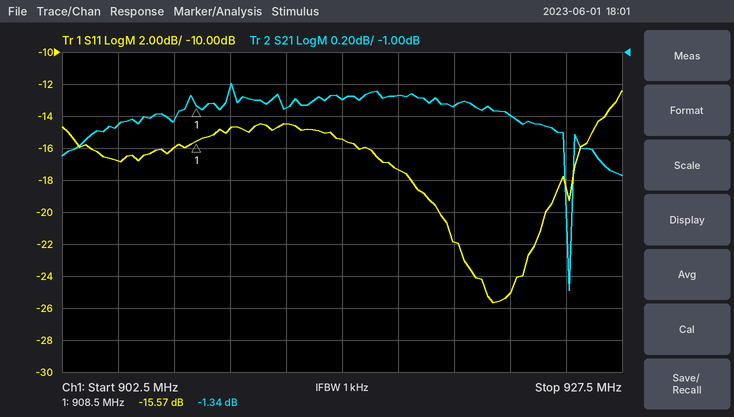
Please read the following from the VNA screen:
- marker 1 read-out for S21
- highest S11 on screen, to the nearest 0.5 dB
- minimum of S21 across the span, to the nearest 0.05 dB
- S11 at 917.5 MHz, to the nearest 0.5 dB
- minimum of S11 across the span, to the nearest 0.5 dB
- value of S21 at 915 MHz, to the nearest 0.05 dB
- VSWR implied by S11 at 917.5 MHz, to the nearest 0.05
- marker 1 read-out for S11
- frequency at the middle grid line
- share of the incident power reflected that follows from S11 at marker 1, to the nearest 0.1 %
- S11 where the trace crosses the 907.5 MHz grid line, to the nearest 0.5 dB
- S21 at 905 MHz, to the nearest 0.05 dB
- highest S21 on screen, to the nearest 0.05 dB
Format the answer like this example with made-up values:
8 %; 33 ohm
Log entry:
-1.34 dB; -12.5 dB; -2.50 dB; -17.5 dB; -25.5 dB; -1.30 dB; 1.30; -15.57 dB; 915 MHz; 2.8 %; -16.0 dB; -1.45 dB; -1.20 dB
